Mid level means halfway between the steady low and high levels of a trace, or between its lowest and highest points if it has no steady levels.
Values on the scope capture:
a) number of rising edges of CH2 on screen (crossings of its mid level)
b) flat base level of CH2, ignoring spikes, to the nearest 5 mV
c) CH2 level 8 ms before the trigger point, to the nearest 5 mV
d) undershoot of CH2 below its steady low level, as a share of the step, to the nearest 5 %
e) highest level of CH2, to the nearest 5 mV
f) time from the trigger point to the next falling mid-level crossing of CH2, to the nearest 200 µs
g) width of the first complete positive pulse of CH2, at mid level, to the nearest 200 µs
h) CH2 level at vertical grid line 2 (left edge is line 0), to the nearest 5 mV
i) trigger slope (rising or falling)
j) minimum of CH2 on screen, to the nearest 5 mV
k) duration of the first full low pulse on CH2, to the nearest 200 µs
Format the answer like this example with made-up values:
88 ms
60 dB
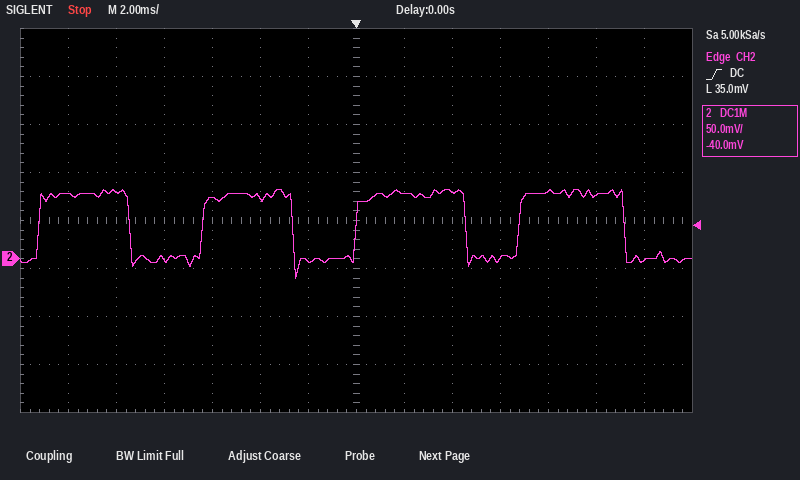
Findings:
4
0 mV
0 mV
30 %
70 mV
4.6 ms
3.8 ms
70 mV
rising
-20 mV
3.0 ms
